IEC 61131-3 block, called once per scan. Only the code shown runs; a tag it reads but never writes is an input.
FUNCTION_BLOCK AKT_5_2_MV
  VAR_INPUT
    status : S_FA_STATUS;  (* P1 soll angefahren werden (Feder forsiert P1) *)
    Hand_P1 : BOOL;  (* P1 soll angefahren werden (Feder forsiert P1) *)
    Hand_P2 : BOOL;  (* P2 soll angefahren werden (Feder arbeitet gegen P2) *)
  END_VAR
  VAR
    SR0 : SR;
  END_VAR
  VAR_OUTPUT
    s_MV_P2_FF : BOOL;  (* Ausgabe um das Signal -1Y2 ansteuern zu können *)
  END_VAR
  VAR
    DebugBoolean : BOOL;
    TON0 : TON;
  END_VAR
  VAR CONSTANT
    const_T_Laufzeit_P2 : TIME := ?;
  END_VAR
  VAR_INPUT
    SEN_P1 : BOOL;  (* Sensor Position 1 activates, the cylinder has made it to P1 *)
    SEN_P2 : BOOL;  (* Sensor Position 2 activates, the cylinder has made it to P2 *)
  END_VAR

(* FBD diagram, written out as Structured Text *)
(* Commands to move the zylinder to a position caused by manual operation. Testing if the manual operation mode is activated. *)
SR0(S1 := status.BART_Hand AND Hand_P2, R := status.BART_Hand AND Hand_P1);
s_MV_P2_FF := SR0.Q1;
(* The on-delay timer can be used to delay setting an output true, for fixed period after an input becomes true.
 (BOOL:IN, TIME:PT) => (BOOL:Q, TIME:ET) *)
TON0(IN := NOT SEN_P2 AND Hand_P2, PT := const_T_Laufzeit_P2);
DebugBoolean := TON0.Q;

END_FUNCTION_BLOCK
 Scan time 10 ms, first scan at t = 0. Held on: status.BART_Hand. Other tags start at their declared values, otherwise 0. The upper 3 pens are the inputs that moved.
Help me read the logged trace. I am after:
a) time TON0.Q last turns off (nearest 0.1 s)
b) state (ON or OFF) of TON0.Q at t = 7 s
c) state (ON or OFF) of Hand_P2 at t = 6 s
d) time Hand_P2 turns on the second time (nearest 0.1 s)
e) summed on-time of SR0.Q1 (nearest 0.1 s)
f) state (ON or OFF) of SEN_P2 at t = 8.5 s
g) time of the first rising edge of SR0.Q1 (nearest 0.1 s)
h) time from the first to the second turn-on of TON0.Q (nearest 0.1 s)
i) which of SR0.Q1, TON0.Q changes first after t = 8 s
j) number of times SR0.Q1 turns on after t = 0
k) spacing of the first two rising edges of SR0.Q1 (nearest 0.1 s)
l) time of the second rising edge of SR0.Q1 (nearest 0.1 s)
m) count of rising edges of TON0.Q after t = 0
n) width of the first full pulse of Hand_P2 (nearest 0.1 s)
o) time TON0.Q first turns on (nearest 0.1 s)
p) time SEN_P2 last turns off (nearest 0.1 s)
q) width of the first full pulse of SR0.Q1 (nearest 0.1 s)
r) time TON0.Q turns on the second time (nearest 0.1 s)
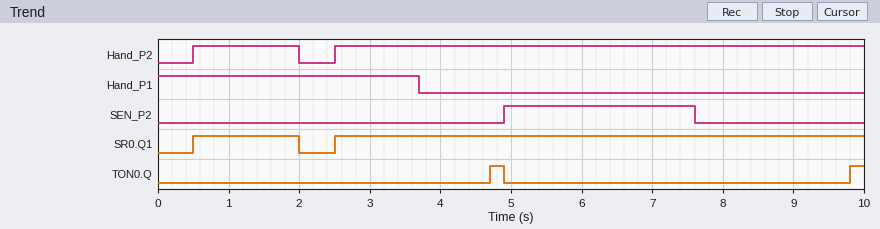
4.9 s
OFF
ON
2.5 s
9.0 s
OFF
0.5 s
5.1 s
TON0.Q
2
2.0 s
2.5 s
2
1.5 s
4.7 s
7.6 s
1.5 s
9.8 s
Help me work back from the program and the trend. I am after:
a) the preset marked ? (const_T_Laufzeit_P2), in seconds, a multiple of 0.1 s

2.2 s
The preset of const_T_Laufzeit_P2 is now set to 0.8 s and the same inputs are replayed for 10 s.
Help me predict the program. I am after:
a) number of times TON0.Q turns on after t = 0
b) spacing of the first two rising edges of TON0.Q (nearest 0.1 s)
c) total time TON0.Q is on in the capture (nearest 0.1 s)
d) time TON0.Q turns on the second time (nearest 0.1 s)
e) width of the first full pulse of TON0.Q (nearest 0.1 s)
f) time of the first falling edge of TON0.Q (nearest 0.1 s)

3
2.0 s
3.9 s
3.3 s
0.7 s
2.0 s
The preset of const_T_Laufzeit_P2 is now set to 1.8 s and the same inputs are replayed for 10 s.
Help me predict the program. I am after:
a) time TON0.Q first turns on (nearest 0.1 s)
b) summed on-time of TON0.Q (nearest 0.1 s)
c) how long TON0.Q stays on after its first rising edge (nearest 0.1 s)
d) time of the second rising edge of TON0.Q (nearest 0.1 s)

4.3 s
1.2 s
0.6 s
9.4 s
